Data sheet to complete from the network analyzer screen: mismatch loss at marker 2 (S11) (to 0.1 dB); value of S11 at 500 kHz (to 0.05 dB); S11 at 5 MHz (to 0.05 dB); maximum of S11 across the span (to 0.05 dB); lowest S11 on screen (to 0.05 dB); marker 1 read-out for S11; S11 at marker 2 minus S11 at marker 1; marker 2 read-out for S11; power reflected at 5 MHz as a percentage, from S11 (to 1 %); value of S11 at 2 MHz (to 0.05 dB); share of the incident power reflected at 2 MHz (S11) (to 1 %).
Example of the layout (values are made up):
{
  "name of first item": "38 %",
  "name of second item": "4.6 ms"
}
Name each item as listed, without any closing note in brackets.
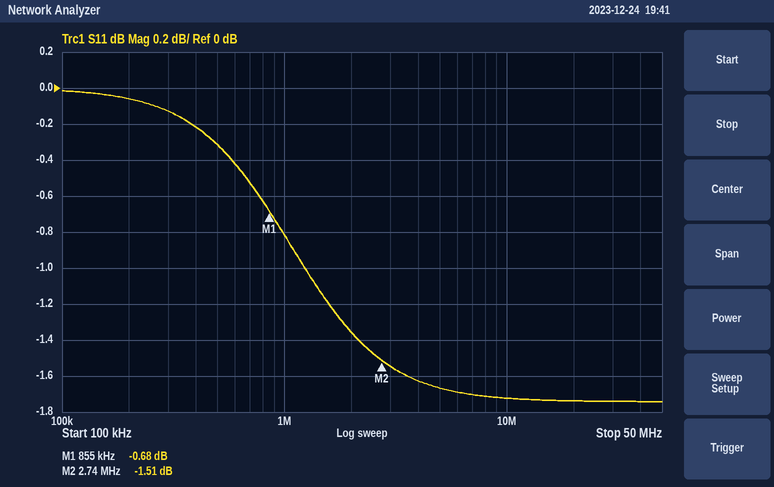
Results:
{
  "mismatch loss at marker 2 (S11)": "5.3 dB",
  "value of S11 at 500 kHz": "-0.30 dB",
  "S11 at 5 MHz": "-1.65 dB",
  "maximum of S11 across the span": "0.00 dB",
  "lowest S11 on screen": "-1.75 dB",
  "marker 1 read-out for S11": "-0.68 dB",
  "S11 at marker 2 minus S11 at marker 1": "-0.83 dB",
  "marker 2 read-out for S11": "-1.51 dB",
  "power reflected at 5 MHz as a percentage, from S11": "68 %",
  "value of S11 at 2 MHz": "-1.35 dB",
  "share of the incident power reflected at 2 MHz (S11)": "73 %"
}
